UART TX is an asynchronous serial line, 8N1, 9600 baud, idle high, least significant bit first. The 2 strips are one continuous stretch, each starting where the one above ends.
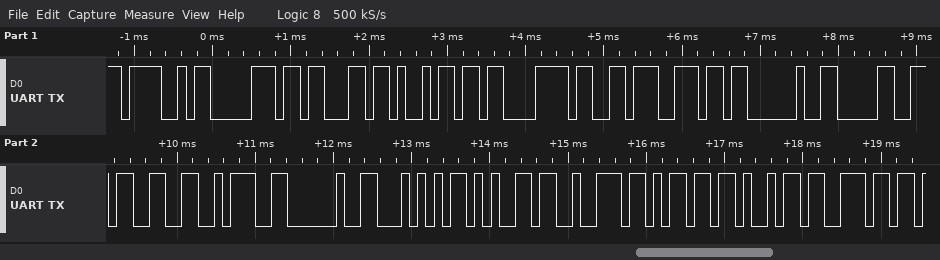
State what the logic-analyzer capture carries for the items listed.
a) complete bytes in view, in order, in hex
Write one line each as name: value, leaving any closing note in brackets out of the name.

complete bytes in view, in order, in hex: 4F 70 63 69 C3 B3 6E 20 30 33 3A 20 54 65 72 6D 69 6E
